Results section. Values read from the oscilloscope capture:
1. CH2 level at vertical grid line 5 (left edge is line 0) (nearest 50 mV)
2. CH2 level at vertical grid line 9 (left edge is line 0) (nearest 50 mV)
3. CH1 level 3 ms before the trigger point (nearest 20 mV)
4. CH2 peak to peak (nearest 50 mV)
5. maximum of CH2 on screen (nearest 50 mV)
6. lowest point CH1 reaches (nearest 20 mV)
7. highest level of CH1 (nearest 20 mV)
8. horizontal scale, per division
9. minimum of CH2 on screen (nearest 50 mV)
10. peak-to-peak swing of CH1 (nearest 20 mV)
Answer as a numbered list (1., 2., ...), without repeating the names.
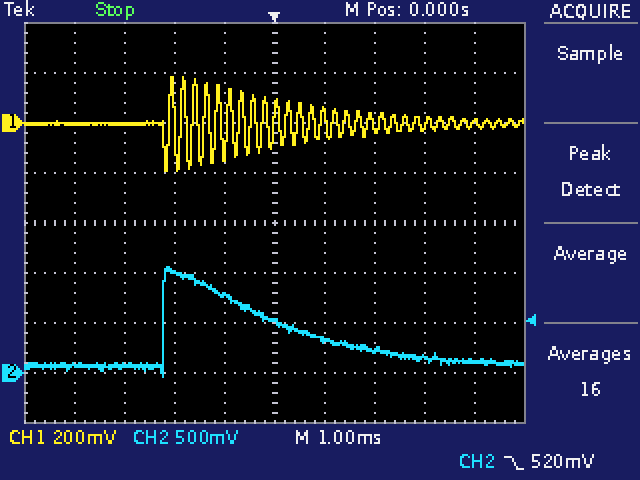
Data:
1. 500 mV
2. 100 mV
3. 0 mV
4. 1.10 V
5. 1.05 V
6. -200 mV
7. 180 mV
8. 1 ms
9. -50 mV
10. 380 mV
